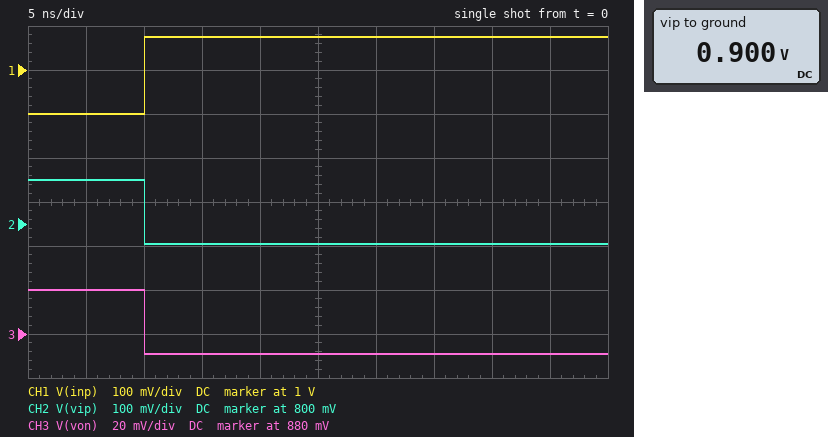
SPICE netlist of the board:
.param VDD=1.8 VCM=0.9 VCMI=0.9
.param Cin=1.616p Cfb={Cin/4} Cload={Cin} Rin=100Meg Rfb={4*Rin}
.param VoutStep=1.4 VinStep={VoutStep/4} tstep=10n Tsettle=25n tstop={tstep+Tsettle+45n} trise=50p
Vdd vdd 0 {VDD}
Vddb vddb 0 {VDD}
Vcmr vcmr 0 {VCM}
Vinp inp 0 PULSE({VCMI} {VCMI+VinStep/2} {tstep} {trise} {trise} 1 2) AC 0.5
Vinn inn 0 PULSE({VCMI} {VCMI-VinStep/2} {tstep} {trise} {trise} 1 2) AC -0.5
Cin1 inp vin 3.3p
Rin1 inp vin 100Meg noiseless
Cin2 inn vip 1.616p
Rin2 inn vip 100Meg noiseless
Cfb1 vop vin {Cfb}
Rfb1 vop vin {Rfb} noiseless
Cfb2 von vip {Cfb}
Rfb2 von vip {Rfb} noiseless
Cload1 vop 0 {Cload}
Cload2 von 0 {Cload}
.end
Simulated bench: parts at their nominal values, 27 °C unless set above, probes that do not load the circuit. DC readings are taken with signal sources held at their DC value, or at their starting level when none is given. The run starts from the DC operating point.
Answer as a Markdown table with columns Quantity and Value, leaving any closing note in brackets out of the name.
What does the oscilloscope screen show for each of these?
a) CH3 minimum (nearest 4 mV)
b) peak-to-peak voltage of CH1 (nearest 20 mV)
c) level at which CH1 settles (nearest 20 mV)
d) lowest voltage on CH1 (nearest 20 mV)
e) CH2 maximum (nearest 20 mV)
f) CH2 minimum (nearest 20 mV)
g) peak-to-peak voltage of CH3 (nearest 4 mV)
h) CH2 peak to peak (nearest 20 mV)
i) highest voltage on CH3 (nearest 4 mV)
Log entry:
| Quantity | Value |
|---|---|
| CH3 minimum | 872 mV |
| peak-to-peak voltage of CH1 | 180 mV |
| level at which CH1 settles | 1.08 V |
| lowest voltage on CH1 | 900 mV |
| CH2 maximum | 900 mV |
| CH2 minimum | 760 mV |
| peak-to-peak voltage of CH3 | 28 mV |
| CH2 peak to peak | 140 mV |
| highest voltage on CH3 | 900 mV |
